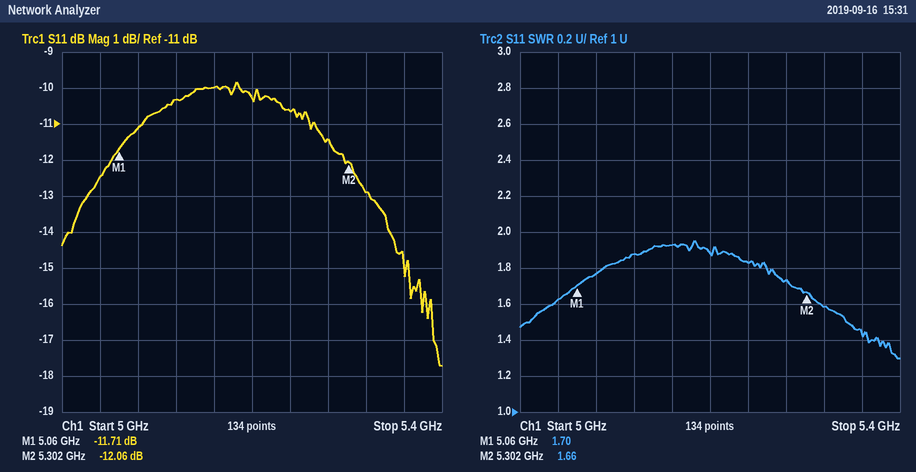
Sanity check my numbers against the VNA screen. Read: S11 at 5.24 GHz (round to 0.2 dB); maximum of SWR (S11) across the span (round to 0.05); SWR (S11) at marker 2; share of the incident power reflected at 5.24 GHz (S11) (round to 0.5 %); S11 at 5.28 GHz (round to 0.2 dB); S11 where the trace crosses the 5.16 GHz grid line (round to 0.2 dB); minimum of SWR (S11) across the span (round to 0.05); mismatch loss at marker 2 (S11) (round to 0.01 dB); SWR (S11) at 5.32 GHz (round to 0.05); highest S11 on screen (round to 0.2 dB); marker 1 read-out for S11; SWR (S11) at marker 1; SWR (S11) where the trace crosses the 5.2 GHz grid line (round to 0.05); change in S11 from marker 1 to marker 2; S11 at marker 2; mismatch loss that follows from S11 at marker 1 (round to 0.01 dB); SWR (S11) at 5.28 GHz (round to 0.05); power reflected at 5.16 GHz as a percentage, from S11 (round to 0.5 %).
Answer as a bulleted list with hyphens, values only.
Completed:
- -10.6 dB
- 1.95
- 1.66
- 8.5 %
- -11.4 dB
- -10.0 dB
- 1.30
- 0.28 dB
- 1.60
- -9.8 dB
- -11.71 dB
- 1.70
- 1.90
- -0.35 dB
- -12.06 dB
- 0.30 dB
- 1.75
- 10.0 %
